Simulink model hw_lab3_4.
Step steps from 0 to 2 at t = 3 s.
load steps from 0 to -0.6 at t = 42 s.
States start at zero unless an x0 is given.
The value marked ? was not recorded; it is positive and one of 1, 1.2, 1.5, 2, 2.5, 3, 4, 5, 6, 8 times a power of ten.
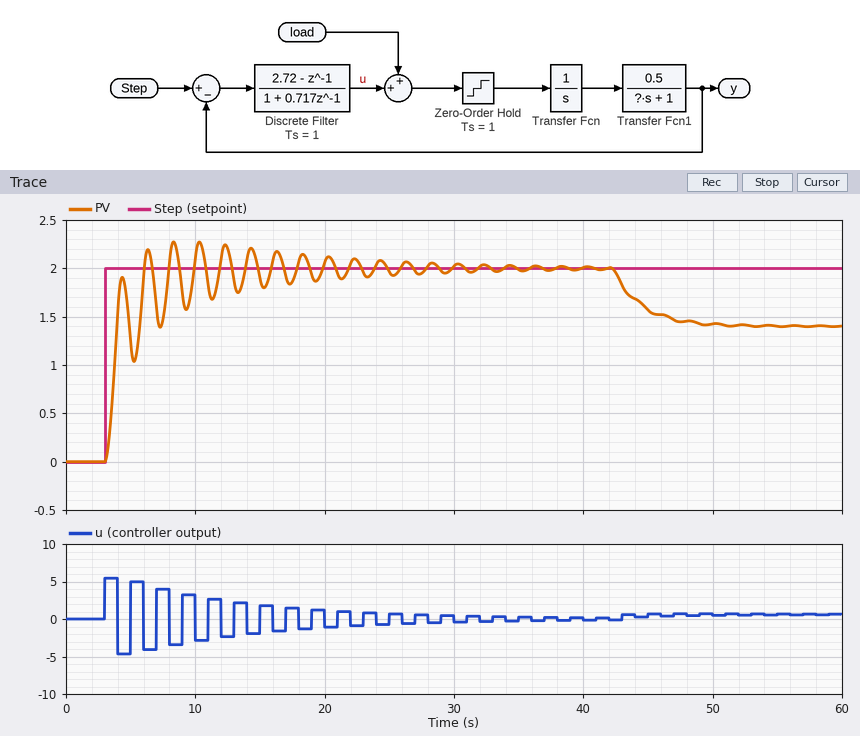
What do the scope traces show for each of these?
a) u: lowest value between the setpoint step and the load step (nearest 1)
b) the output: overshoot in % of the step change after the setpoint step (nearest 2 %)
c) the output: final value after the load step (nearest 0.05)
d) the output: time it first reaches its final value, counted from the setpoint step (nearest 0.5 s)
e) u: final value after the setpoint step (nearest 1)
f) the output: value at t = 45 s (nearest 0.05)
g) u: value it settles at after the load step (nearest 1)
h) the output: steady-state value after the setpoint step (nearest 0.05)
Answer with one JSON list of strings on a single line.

["-5", "14 %", "1.40", "3.0 s", "0", "1.55", "1", "2.00"]
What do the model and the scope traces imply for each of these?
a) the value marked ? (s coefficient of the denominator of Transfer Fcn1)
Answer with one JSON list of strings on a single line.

["0.5"]
